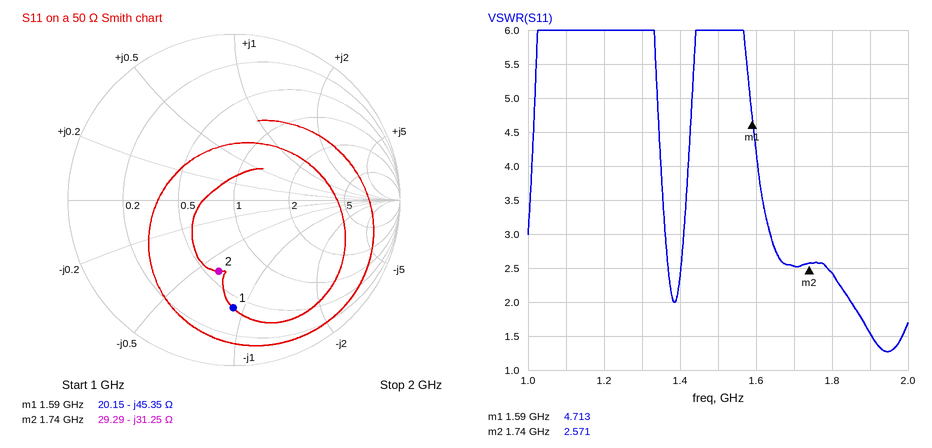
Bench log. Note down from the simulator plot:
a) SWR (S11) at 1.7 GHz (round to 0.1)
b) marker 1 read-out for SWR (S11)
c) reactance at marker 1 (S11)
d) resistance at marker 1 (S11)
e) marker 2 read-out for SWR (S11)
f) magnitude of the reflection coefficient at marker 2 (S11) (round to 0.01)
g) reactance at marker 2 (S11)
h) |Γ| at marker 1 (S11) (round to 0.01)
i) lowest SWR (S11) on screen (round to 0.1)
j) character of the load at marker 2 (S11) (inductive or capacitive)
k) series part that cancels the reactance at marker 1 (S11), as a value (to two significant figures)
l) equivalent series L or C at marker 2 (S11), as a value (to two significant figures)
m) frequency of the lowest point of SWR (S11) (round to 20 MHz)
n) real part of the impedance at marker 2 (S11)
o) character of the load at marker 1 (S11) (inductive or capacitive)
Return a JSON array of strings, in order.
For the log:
["2.5", "4.713", "-45.35 Ω", "20.15 Ω", "2.571", "0.44", "-31.25 Ω", "0.65", "1.3", "capacitive", "4.5 nH", "2.9 pF", "1.94 GHz", "29.29 Ω", "capacitive"]
